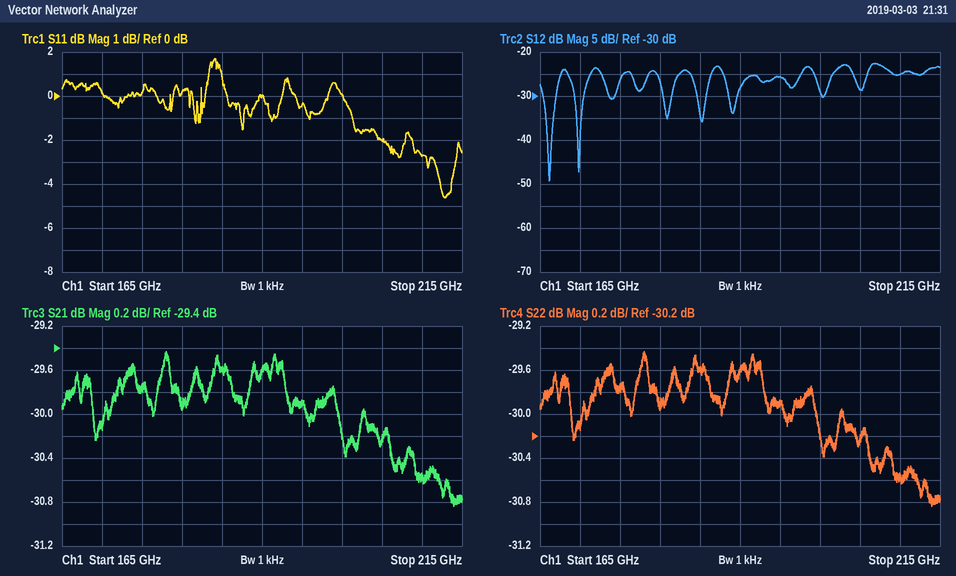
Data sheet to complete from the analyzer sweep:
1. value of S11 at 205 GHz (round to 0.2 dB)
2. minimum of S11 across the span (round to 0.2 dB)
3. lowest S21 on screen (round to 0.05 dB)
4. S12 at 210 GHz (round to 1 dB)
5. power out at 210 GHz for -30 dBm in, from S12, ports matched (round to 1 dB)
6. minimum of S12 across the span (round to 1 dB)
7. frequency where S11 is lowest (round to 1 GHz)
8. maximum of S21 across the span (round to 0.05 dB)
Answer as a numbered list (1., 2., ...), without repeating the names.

1. -2.0 dB
2. -4.6 dB
3. -30.85 dB
4. -25 dB
5. -55 dBm
6. -49 dB
7. 213 GHz
8. -29.45 dB
